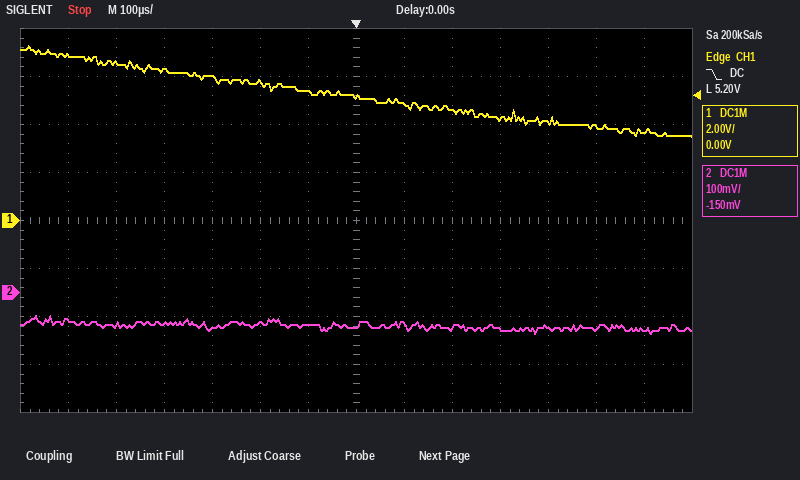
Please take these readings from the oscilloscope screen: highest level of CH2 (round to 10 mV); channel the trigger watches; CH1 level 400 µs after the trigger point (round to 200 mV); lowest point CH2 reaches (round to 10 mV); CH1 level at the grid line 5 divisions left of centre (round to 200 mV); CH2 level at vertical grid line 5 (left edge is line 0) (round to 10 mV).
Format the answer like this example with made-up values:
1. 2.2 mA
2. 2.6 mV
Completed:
1. -50 mV
2. CH1
3. 4.0 V
4. -90 mV
5. 6.6 V
6. -60 mV
